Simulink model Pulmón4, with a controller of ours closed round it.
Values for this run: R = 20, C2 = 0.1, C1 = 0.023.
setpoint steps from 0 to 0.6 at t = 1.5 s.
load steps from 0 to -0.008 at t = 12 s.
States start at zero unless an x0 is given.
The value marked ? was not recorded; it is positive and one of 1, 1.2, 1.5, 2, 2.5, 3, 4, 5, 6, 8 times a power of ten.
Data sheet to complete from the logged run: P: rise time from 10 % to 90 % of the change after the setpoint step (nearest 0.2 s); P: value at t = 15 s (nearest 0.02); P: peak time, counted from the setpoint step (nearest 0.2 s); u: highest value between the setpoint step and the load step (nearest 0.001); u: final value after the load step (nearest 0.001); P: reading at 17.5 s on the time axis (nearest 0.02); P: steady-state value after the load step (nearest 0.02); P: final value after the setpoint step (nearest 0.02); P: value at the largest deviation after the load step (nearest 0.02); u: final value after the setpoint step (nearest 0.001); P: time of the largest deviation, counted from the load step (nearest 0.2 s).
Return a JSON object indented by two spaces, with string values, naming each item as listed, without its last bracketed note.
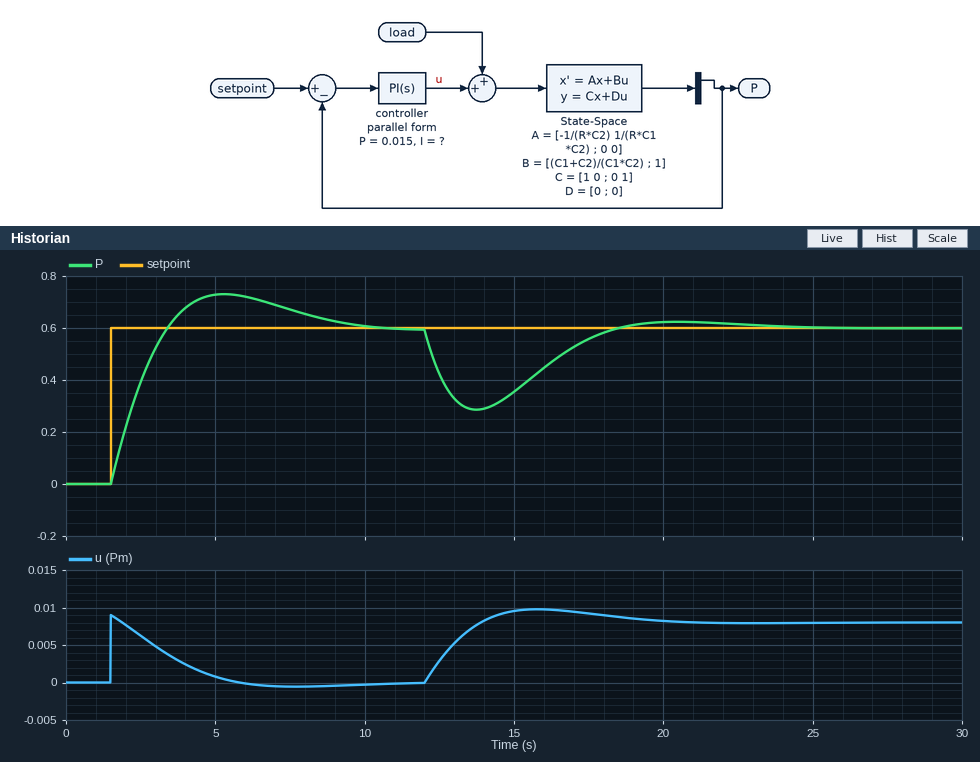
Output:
{
  "P: rise time from 10 % to 90 % of the change after the setpoint step": "1.4 s",
  "P: value at t = 15 s": "0.36",
  "P: peak time, counted from the setpoint step": "3.8 s",
  "u: highest value between the setpoint step and the load step": "0.009",
  "u: final value after the load step": "0.008",
  "P: reading at 17.5 s on the time axis": "0.56",
  "P: steady-state value after the load step": "0.60",
  "P: final value after the setpoint step": "0.60",
  "P: value at the largest deviation after the load step": "0.28",
  "u: final value after the setpoint step": "0.000",
  "P: time of the largest deviation, counted from the load step": "1.8 s"
}
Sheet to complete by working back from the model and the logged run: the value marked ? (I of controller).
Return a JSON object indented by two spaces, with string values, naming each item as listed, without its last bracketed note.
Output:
{
  "the value marked ?": "0.008"
}
